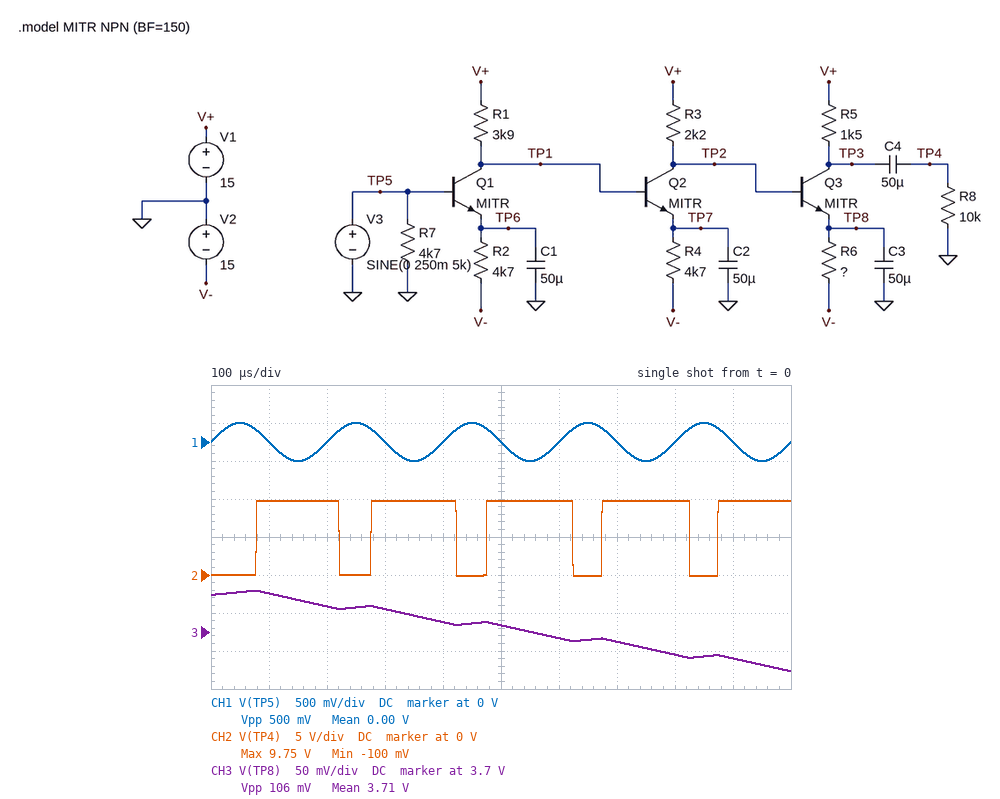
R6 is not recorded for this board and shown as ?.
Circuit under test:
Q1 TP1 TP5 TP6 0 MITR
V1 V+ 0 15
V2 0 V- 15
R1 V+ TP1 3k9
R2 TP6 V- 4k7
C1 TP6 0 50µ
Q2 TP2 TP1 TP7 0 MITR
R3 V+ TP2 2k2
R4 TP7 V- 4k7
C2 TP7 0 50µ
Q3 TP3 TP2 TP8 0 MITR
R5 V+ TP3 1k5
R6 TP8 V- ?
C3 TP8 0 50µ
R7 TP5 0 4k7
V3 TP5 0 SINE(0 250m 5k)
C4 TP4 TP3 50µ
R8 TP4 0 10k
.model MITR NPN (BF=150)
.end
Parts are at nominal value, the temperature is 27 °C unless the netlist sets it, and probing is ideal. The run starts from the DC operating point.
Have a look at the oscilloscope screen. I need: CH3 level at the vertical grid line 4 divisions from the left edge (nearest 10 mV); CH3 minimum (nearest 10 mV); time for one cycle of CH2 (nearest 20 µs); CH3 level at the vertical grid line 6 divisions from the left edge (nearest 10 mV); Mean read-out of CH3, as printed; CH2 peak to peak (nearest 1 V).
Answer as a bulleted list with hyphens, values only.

- 3.71 V
- 3.65 V
- 200 µs
- 3.69 V
- 3.71 V
- 10 V
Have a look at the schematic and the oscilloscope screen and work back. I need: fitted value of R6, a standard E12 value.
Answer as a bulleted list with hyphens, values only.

- 2.2 kΩ
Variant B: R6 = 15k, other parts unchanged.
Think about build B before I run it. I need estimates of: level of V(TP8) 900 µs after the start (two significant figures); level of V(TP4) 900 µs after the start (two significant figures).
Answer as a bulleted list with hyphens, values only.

- 6.1 V
- 1.8 V
